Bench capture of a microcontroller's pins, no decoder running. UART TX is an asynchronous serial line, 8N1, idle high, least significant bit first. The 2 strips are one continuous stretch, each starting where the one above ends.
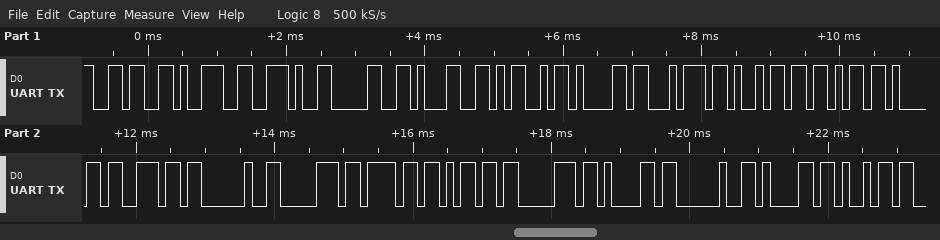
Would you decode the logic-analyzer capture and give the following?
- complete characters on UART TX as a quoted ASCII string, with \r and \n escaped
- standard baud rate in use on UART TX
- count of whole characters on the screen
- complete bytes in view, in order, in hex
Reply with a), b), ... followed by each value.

a) "69.01Matikan pompa ai"
b) 9600 baud
c) 21
d) 36 39 2E 30 31 4D 61 74 69 6B 61 6E 20 70 6F 6D 70 61 20 61 69
